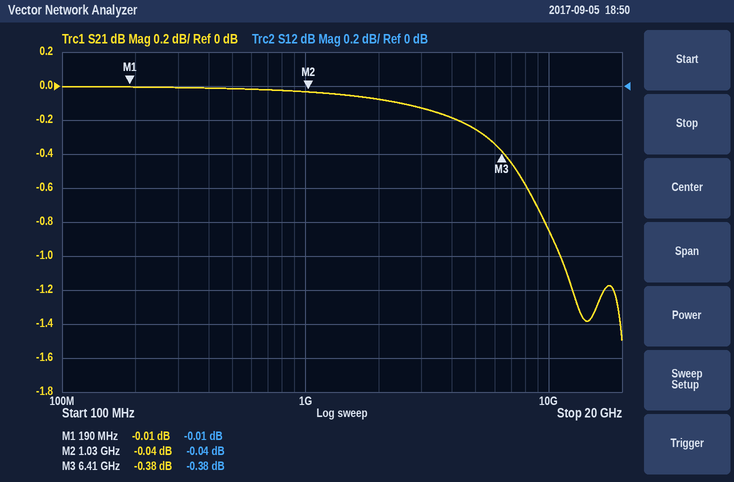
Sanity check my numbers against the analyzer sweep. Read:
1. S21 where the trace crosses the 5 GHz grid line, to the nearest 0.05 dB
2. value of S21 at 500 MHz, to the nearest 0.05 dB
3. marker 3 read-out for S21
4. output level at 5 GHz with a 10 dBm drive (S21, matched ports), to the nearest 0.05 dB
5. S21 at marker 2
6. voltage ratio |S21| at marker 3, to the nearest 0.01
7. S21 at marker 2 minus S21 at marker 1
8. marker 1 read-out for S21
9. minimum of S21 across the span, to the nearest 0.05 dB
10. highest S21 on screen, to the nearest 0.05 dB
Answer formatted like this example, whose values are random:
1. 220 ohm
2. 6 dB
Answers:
1. -0.25 dB
2. 0.00 dB
3. -0.38 dB
4. 9.75 dBm
5. -0.04 dB
6. 0.96
7. -0.03 dB
8. -0.01 dB
9. -1.50 dB
10. 0.00 dB
